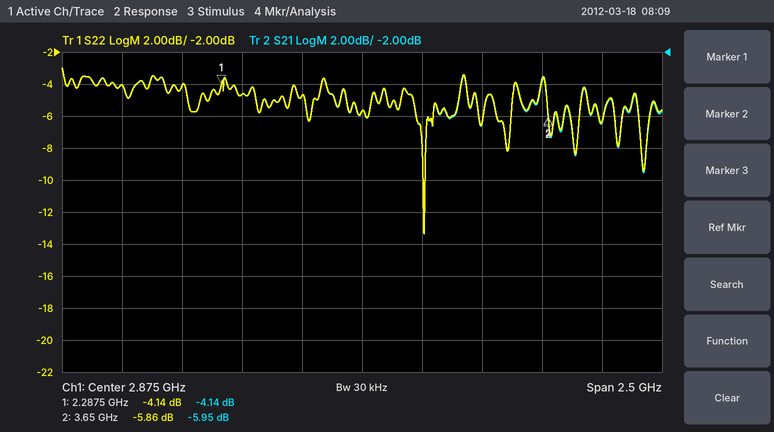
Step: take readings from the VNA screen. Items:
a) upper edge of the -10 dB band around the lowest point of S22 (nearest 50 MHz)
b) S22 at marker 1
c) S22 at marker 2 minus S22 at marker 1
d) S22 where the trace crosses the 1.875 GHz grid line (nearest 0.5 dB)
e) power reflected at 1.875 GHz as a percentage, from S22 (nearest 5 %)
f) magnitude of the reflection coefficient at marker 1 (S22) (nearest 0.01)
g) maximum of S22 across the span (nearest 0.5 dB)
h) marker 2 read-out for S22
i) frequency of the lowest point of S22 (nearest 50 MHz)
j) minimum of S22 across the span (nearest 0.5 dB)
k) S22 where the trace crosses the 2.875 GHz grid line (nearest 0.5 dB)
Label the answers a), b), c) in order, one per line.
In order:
a) 3.15 GHz
b) -4.14 dB
c) -1.72 dB
d) -4.0 dB
e) 40 %
f) 0.62
g) -3.0 dB
h) -5.86 dB
i) 3.15 GHz
j) -13.5 dB
k) -5.5 dB
